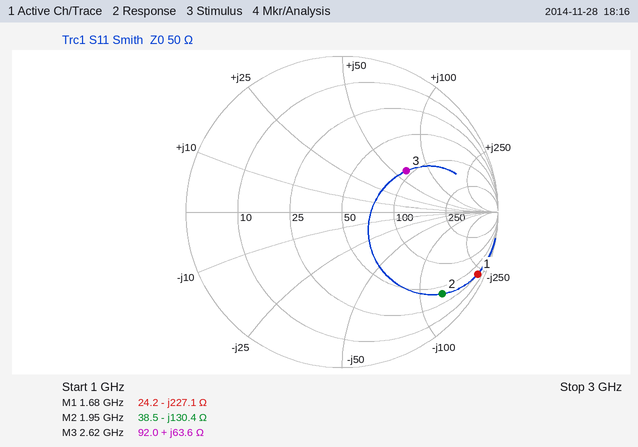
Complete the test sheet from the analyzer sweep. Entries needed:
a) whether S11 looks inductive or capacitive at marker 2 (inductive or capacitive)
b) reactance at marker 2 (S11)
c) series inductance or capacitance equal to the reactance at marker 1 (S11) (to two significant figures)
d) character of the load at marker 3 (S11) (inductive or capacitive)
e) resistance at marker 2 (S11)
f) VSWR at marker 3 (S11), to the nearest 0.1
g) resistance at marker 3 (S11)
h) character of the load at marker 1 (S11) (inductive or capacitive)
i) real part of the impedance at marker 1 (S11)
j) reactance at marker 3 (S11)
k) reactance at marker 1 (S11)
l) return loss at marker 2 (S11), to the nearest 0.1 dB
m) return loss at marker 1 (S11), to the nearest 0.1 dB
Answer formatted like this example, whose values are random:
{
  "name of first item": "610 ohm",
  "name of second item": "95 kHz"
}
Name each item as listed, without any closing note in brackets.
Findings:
{
  "whether S11 looks inductive or capacitive at marker 2": "capacitive",
  "reactance at marker 2": "-130.4 Ω",
  "series inductance or capacitance equal to the reactance at marker 1 (S11)": "420 fF",
  "character of the load at marker 3 (S11)": "inductive",
  "resistance at marker 2": "38.5 Ω",
  "VSWR at marker 3 (S11), to the nearest 0.1": "2.9",
  "resistance at marker 3": "92.0 Ω",
  "character of the load at marker 1 (S11)": "capacitive",
  "real part of the impedance at marker 1": "24.2 Ω",
  "reactance at marker 3": "+63.6 Ω",
  "reactance at marker 1": "-227.1 Ω",
  "return loss at marker 2 (S11), to the nearest 0.1 dB": "1.6 dB",
  "return loss at marker 1 (S11), to the nearest 0.1 dB": "0.4 dB"
}
